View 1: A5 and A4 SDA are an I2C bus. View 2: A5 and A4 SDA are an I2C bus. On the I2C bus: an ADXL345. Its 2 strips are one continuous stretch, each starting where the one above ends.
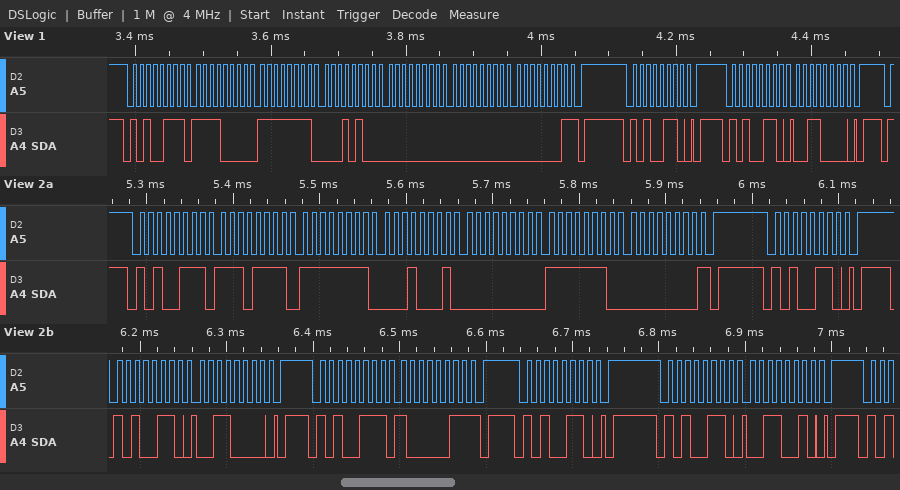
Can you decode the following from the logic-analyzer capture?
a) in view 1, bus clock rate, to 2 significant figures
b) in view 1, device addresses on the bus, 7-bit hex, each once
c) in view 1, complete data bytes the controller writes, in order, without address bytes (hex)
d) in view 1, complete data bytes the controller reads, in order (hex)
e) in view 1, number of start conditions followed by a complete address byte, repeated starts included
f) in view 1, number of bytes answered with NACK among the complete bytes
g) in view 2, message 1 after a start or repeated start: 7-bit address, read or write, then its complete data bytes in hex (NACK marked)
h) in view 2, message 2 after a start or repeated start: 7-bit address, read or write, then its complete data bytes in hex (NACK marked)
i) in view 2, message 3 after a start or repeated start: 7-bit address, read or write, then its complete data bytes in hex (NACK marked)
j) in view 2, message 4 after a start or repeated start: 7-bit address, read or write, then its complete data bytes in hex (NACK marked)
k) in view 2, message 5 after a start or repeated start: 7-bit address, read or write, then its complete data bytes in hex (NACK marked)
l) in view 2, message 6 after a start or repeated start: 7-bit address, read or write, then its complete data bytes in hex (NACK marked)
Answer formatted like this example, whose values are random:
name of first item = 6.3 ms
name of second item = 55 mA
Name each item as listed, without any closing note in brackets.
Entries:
in view 1, bus clock rate, to 2 significant figures = 100 kHz
in view 1, device addresses on the bus, 7-bit hex, each once = 0x53
in view 1, complete data bytes the controller writes, in order, without address bytes = 30
in view 1, complete data bytes the controller reads, in order = F0 FF 14 00 00 01
in view 1, number of start conditions followed by a complete address byte, repeated starts included = 3
in view 1, number of bytes answered with NACK among the complete bytes = 1
in view 2, message 1 after a start or repeated start: 7-bit address, read or write, then its complete data bytes in hex = 0x53 read: EF FF 11 00 FE 00 NACK
in view 2, message 2 after a start or repeated start: 7-bit address, read or write, then its complete data bytes in hex = 0x53 write
in view 2, message 3 after a start or repeated start: 7-bit address, read or write, then its complete data bytes in hex = 0x53 write: 30
in view 2, message 4 after a start or repeated start: 7-bit address, read or write, then its complete data bytes in hex = 0x53 read: 83 NACK
in view 2, message 5 after a start or repeated start: 7-bit address, read or write, then its complete data bytes in hex = 0x53 write
in view 2, message 6 after a start or repeated start: 7-bit address, read or write, then its complete data bytes in hex = 0x53 write: 32
